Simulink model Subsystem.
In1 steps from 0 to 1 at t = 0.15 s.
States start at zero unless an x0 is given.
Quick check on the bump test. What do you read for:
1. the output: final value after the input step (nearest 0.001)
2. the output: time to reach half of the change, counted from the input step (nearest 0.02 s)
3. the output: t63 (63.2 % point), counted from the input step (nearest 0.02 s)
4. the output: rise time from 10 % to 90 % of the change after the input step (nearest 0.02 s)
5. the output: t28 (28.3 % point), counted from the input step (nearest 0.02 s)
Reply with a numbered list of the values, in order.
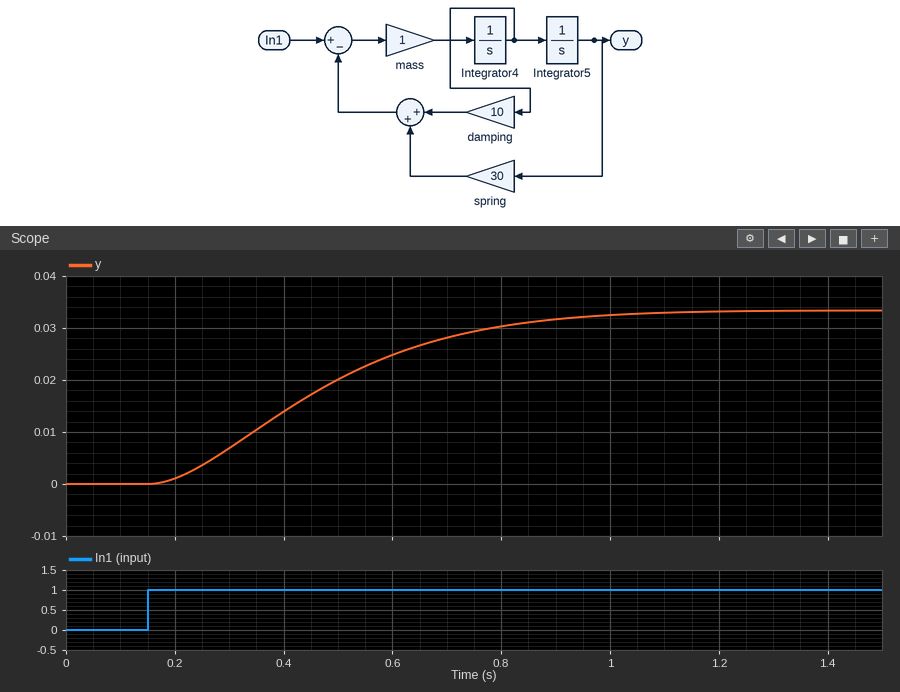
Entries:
1. 0.033
2. 0.30 s
3. 0.36 s
4. 0.54 s
5. 0.18 s
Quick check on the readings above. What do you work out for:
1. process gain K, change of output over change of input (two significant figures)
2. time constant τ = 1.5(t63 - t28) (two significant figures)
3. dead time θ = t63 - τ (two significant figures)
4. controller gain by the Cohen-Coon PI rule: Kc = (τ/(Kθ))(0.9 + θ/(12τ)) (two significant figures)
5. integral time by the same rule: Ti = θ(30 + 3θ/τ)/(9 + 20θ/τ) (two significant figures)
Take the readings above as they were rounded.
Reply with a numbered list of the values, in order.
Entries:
1. 0.033
2. 0.27 s
3. 0.090 s
4. 84
5. 0.18 s
